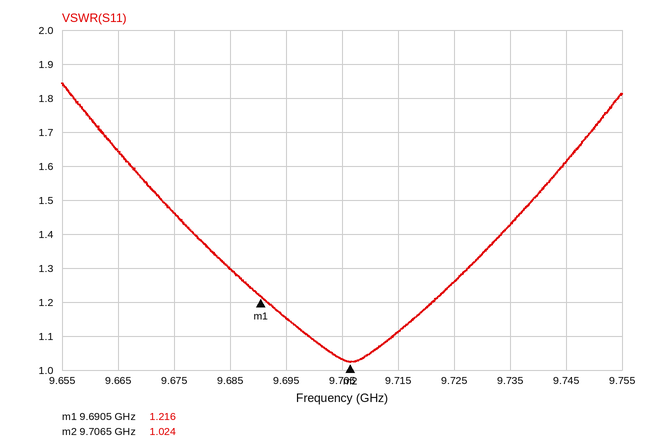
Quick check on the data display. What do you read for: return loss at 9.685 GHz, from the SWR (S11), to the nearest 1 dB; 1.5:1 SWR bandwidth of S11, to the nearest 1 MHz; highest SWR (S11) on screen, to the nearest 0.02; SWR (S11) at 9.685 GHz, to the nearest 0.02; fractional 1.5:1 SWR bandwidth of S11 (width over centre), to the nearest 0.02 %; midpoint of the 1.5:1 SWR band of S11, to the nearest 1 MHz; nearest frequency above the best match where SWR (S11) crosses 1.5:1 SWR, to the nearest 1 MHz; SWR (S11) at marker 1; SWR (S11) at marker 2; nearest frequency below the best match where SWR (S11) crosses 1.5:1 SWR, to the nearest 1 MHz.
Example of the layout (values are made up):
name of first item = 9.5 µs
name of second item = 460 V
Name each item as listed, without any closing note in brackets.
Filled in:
return loss at 9.685 GHz, from the SWR (S11), to the nearest 1 dB = 18 dB
1.5:1 SWR bandwidth of S11, to the nearest 1 MHz = 66 MHz
highest SWR (S11) on screen, to the nearest 0.02 = 1.84
SWR (S11) at 9.685 GHz, to the nearest 0.02 = 1.30
fractional 1.5:1 SWR bandwidth of S11 (width over centre), to the nearest 0.02 % = 0.68 %
midpoint of the 1.5:1 SWR band of S11, to the nearest 1 MHz = 9.706 GHz
nearest frequency above the best match where SWR (S11) crosses 1.5:1 SWR, to the nearest 1 MHz = 9.739 GHz
SWR (S11) at marker 1 = 1.216
SWR (S11) at marker 2 = 1.024
nearest frequency below the best match where SWR (S11) crosses 1.5:1 SWR, to the nearest 1 MHz = 9.673 GHz
